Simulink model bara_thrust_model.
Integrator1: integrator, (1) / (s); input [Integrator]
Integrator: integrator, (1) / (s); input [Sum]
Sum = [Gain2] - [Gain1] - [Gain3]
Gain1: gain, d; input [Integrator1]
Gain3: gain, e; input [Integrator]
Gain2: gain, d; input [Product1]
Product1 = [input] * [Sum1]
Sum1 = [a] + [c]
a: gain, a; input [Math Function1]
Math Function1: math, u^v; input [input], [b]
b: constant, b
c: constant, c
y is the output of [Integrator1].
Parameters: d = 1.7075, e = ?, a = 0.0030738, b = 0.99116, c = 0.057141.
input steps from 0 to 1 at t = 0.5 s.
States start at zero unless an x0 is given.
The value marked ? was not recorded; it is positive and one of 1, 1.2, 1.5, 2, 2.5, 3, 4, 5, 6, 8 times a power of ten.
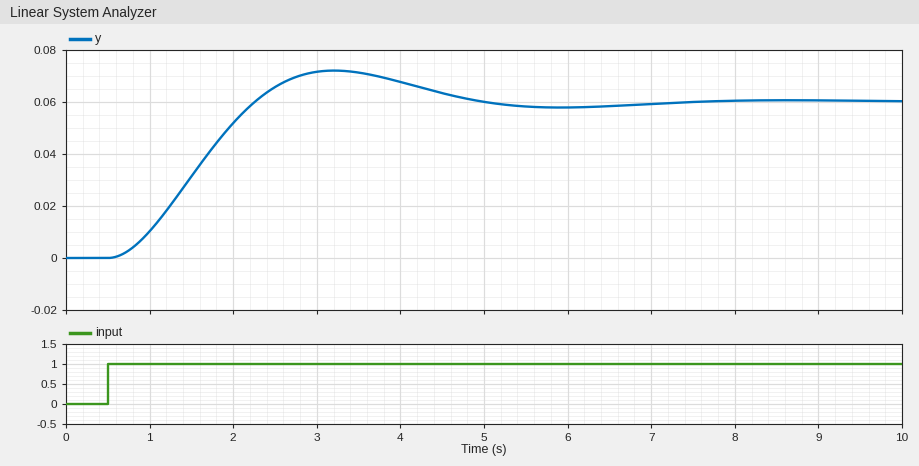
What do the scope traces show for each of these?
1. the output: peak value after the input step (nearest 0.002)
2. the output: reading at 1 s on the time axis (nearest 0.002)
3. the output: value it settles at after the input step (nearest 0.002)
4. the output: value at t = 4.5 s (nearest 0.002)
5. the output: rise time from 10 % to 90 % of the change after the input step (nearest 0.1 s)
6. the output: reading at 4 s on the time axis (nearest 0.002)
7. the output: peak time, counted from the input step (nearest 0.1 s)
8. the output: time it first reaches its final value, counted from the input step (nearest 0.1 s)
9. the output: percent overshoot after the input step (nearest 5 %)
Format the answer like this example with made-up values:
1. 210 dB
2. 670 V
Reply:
1. 0.072
2. 0.010
3. 0.060
4. 0.064
5. 1.2 s
6. 0.068
7. 2.7 s
8. 1.8 s
9. 20 %
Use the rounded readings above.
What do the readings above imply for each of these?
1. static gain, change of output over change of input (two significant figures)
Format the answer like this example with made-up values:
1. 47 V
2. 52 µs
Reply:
1. 0.060
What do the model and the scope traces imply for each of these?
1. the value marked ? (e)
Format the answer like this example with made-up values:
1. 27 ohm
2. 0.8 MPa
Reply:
1. 1.2
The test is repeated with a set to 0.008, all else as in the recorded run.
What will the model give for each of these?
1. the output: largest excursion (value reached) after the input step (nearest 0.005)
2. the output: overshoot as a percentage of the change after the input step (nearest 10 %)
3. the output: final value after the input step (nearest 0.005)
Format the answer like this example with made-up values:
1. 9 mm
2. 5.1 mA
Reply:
1. 0.080
2. 20 %
3. 0.065
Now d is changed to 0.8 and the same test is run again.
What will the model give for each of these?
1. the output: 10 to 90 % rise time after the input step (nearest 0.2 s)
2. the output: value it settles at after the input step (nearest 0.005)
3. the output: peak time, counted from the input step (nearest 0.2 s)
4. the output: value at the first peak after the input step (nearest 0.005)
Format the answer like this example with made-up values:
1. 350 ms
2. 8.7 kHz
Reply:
1. 2.2 s
2. 0.060
3. 4.8 s
4. 0.065
